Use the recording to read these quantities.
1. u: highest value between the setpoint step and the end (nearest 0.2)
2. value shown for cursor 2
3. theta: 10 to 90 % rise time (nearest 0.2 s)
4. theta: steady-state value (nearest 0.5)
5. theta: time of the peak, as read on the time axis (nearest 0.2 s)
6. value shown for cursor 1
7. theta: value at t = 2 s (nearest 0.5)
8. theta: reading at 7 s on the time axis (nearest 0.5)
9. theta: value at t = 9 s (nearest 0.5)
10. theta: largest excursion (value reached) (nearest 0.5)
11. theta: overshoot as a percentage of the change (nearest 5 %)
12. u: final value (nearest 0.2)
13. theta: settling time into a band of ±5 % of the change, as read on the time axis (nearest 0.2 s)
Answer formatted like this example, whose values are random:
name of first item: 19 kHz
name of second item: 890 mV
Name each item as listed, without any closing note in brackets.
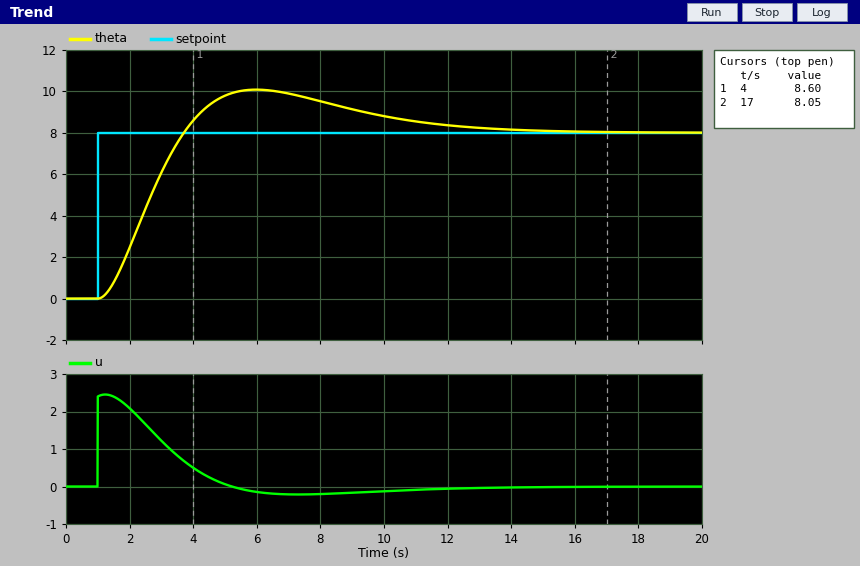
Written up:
u: highest value between the setpoint step and the end: 2.4
value shown for cursor 2: 8.05
theta: 10 to 90 % rise time: 1.8 s
theta: steady-state value: 8.0
theta: time of the peak, as read on the time axis: 6.0 s
value shown for cursor 1: 8.60
theta: value at t = 2 s: 2.5
theta: reading at 7 s on the time axis: 10.0
theta: value at t = 9 s: 9.0
theta: largest excursion (value reached): 10.0
theta: overshoot as a percentage of the change: 25 %
u: final value: 0.0
theta: settling time into a band of ±5 % of the change, as read on the time axis: 11.8 s
